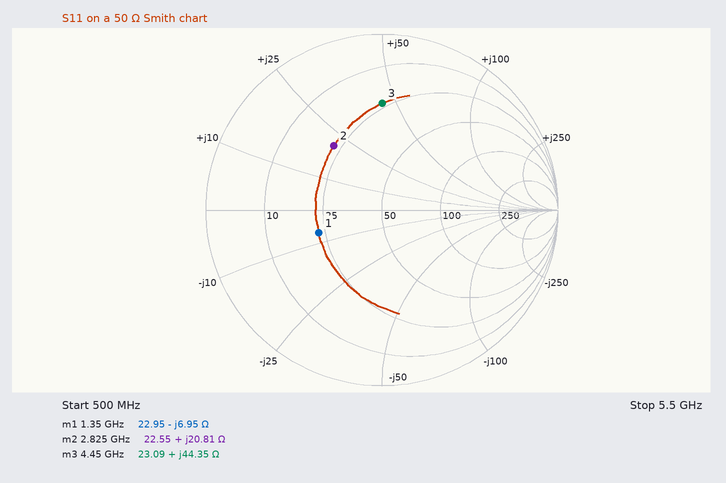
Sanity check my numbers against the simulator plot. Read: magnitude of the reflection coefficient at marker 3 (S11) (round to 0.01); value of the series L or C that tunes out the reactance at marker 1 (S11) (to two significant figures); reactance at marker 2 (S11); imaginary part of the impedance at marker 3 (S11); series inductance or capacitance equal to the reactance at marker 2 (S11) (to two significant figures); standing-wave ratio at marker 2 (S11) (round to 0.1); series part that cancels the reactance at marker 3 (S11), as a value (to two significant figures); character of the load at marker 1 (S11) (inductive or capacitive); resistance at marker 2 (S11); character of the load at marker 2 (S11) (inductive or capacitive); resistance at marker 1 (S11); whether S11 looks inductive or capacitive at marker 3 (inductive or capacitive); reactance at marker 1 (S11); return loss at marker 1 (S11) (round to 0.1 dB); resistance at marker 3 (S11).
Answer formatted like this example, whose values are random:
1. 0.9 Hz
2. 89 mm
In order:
1. 0.61
2. 820 pH
3. +20.81 Ω
4. +44.35 Ω
5. 1.2 nH
6. 2.7
7. 810 fF
8. capacitive
9. 22.55 Ω
10. inductive
11. 22.95 Ω
12. inductive
13. -6.95 Ω
14. 8.4 dB
15. 23.09 Ω
